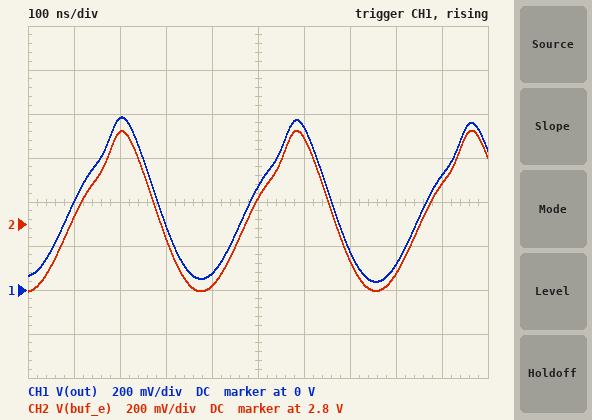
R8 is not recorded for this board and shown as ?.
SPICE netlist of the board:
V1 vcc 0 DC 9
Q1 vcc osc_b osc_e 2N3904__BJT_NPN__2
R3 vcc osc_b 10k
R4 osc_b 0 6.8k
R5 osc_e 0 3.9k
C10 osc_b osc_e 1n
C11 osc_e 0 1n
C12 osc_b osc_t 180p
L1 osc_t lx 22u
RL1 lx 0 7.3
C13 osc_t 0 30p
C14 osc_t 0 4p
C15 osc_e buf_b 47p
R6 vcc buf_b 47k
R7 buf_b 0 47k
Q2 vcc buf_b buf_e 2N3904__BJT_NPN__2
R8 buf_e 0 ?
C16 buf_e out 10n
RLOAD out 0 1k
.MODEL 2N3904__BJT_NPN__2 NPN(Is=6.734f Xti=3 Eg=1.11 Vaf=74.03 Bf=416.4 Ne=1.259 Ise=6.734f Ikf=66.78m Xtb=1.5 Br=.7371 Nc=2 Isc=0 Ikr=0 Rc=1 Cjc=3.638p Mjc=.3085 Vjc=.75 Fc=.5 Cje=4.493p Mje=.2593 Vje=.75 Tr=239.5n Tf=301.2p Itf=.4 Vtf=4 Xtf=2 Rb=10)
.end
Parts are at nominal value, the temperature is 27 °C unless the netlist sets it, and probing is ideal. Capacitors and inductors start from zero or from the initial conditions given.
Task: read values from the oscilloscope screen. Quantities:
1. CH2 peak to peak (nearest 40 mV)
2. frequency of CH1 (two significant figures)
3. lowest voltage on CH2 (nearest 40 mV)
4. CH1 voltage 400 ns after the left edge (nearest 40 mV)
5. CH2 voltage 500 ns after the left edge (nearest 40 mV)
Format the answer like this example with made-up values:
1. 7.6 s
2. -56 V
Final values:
1. 720 mV
2. 2.6 MHz
3. 2.48 V
4. 80 mV
5. 2.92 V
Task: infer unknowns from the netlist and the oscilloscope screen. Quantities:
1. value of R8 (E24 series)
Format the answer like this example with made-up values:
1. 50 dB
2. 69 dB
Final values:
1. 430 Ω
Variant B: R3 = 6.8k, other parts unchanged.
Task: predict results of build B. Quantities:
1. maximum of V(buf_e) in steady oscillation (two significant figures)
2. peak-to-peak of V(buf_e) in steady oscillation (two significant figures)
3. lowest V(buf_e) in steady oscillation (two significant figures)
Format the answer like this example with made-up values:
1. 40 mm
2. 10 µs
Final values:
1. 3.3 V
2. 930 mV
3. 2.4 V
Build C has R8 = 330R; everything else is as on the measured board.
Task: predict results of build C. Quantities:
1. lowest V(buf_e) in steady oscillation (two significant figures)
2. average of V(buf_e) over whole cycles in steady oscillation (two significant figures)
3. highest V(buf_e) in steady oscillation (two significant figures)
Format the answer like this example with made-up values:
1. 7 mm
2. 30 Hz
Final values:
1. 2.3 V
2. 2.6 V
3. 3.0 V
